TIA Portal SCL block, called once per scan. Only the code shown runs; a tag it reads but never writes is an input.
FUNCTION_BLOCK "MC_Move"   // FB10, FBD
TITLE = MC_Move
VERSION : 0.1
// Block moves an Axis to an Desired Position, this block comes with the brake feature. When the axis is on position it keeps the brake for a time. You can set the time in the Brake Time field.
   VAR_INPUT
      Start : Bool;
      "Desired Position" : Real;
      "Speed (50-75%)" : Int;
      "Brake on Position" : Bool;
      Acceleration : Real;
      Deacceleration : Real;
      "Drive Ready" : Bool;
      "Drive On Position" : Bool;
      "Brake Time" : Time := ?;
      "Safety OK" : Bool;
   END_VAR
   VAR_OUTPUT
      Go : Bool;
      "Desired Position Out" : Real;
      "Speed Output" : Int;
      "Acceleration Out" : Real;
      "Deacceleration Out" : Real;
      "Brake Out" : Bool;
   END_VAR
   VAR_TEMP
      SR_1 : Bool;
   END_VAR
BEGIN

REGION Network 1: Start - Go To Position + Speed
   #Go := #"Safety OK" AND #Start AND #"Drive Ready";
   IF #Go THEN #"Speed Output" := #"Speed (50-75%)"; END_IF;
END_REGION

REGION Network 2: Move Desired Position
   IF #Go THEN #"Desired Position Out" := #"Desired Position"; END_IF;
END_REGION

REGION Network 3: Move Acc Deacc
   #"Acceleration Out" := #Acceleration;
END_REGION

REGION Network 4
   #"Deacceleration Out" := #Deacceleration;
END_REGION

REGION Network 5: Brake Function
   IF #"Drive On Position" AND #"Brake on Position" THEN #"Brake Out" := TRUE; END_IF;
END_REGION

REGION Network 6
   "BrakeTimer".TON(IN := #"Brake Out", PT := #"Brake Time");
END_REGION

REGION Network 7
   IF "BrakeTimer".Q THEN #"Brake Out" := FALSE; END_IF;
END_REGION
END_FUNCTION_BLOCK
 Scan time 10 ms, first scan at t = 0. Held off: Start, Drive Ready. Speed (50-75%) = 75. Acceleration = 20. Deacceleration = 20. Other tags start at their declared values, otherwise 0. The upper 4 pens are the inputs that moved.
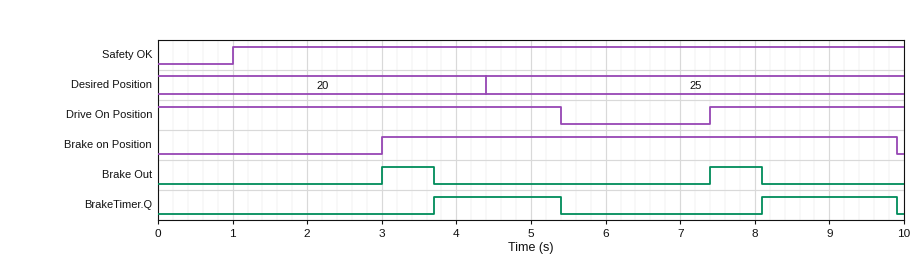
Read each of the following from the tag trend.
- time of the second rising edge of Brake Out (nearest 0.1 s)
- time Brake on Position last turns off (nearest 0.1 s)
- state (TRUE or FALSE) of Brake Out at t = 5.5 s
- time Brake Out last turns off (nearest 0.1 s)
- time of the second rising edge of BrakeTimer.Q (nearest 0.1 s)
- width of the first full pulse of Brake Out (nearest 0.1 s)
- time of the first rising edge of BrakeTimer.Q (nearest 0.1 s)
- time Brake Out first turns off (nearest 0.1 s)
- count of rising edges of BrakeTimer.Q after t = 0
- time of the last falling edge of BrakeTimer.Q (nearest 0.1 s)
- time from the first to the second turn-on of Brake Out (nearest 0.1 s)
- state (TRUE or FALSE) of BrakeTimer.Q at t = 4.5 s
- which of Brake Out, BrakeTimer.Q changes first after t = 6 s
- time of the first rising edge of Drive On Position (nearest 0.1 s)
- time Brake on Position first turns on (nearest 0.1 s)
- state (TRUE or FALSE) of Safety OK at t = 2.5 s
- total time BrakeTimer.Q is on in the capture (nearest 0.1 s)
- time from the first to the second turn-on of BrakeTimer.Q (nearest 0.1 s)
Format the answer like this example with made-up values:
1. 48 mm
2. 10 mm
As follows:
1. 7.4 s
2. 9.9 s
3. FALSE
4. 8.1 s
5. 8.1 s
6. 0.7 s
7. 3.7 s
8. 3.7 s
9. 2
10. 9.9 s
11. 4.4 s
12. TRUE
13. Brake Out
14. 7.4 s
15. 3.0 s
16. TRUE
17. 3.5 s
18. 4.4 s
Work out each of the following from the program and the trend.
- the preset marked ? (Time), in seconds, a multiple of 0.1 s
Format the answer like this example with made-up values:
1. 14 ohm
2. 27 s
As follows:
1. 0.7 s
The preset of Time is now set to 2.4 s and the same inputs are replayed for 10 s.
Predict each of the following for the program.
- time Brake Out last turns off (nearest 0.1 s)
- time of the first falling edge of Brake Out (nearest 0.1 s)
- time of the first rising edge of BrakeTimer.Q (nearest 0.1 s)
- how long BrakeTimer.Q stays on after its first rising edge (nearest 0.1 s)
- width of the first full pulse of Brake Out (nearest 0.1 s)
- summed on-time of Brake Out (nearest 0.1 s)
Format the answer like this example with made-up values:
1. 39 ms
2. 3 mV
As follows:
1. 9.8 s
2. 5.4 s
3. 5.4 s
4. 0.0 s
5. 2.4 s
6. 4.8 s
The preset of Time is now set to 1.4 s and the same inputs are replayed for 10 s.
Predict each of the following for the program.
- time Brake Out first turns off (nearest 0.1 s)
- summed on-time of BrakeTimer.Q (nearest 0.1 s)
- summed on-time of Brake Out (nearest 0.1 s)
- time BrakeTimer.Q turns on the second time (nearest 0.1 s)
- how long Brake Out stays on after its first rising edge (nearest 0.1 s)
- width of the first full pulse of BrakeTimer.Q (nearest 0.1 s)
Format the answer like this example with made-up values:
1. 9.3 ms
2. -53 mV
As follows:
1. 4.4 s
2. 2.1 s
3. 2.8 s
4. 8.8 s
5. 1.4 s
6. 1.0 s
